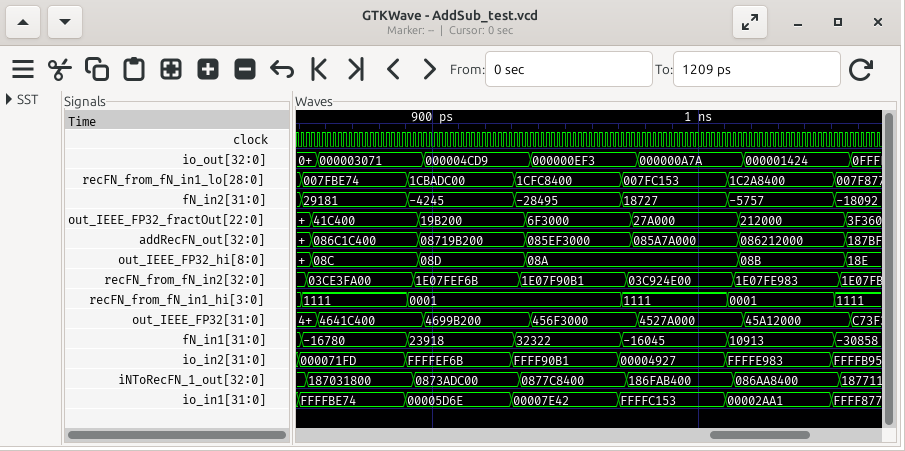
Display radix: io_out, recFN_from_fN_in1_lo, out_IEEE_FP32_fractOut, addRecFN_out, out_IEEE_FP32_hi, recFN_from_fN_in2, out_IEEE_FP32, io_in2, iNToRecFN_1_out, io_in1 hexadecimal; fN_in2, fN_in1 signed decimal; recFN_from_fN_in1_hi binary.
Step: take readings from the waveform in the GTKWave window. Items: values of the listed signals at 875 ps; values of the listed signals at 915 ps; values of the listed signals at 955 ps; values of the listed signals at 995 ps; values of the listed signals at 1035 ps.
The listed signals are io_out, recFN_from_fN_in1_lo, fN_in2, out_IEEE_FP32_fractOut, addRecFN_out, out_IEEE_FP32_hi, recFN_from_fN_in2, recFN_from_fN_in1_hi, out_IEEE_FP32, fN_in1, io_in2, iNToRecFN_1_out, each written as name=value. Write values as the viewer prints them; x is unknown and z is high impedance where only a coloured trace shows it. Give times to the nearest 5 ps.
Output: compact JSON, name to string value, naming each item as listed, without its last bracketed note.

{"values of the listed signals at 875 ps": "io_out=000003071, recFN_from_fN_in1_lo=007FBE74, fN_in2=29181, out_IEEE_FP32_fractOut=41C400, addRecFN_out=086C1C400, out_IEEE_FP32_hi=08C, recFN_from_fN_in2=03CE3FA00, recFN_from_fN_in1_hi=1111, out_IEEE_FP32=4641C400, fN_in1=-16780, io_in2=000071FD, iNToRecFN_1_out=187031800", "values of the listed signals at 915 ps": "io_out=000004CD9, recFN_from_fN_in1_lo=1CBADC00, fN_in2=-4245, out_IEEE_FP32_fractOut=19B200, addRecFN_out=08719B200, out_IEEE_FP32_hi=08D, recFN_from_fN_in2=1E07FEF6B, recFN_from_fN_in1_hi=0001, out_IEEE_FP32=4699B200, fN_in1=23918, io_in2=FFFFEF6B, iNToRecFN_1_out=0873ADC00", "values of the listed signals at 955 ps": "io_out=000000EF3, recFN_from_fN_in1_lo=1CFC8400, fN_in2=-28495, out_IEEE_FP32_fractOut=6F3000, addRecFN_out=085EF3000, out_IEEE_FP32_hi=08A, recFN_from_fN_in2=1E07F90B1, recFN_from_fN_in1_hi=0001, out_IEEE_FP32=456F3000, fN_in1=32322, io_in2=FFFF90B1, iNToRecFN_1_out=0877C8400", "values of the listed signals at 995 ps": "io_out=000000A7A, recFN_from_fN_in1_lo=007FC153, fN_in2=18727, out_IEEE_FP32_fractOut=27A000, addRecFN_out=085A7A000, out_IEEE_FP32_hi=08A, recFN_from_fN_in2=03C924E00, recFN_from_fN_in1_hi=1111, out_IEEE_FP32=4527A000, fN_in1=-16045, io_in2=00004927, iNToRecFN_1_out=186FAB400", "values of the listed signals at 1035 ps": "io_out=000001424, recFN_from_fN_in1_lo=1C2A8400, fN_in2=-5757, out_IEEE_FP32_fractOut=212000, addRecFN_out=086212000, out_IEEE_FP32_hi=08B, recFN_from_fN_in2=1E07FE983, recFN_from_fN_in1_hi=0001, out_IEEE_FP32=45A12000, fN_in1=10913, io_in2=FFFFE983, iNToRecFN_1_out=086AA8400"}
